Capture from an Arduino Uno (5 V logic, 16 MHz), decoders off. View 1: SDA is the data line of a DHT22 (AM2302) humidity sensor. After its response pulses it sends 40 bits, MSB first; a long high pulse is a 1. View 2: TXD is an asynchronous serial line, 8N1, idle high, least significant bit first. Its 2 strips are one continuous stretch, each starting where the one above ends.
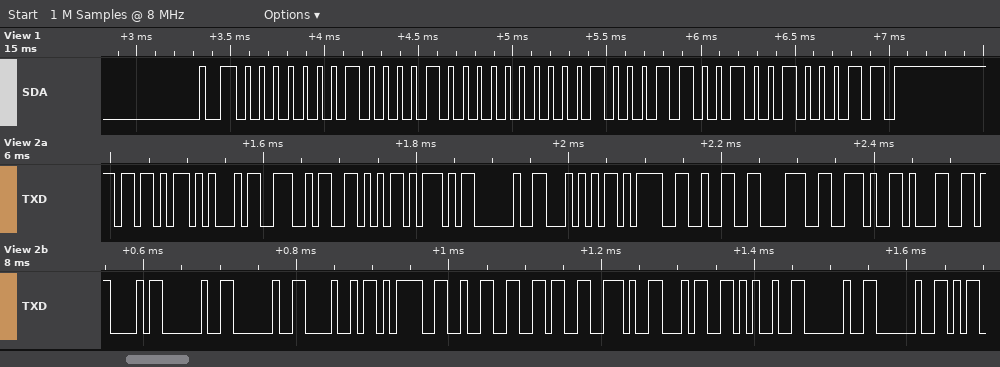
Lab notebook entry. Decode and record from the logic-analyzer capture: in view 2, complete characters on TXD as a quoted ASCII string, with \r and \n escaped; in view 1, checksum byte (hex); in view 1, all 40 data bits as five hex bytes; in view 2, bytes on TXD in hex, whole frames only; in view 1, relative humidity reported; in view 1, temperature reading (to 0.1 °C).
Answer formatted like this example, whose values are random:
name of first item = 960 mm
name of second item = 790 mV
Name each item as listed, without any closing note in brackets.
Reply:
in view 2, complete characters on TXD as a quoted ASCII string, with \r and \n escaped = "[ENV] T=28.1C  H=26.4%  "
in view 1, checksum byte = 0x23
in view 1, all 40 data bits as five hex bytes = 01 08 01 19 23
in view 2, bytes on TXD in hex, whole frames only = 5B 45 4E 56 5D 20 54 3D 32 38 2E 31 43 20 20 48 3D 32 36 2E 34 25 20 20
in view 1, relative humidity reported = 26.4 %
in view 1, temperature reading = 28.1 °C
